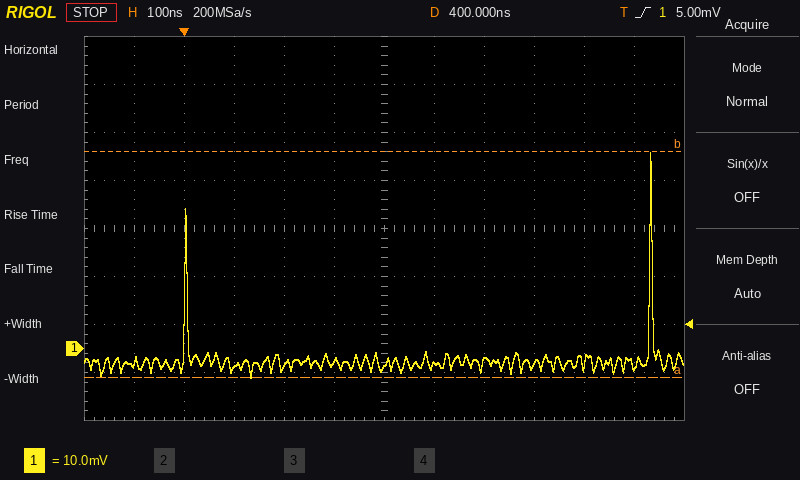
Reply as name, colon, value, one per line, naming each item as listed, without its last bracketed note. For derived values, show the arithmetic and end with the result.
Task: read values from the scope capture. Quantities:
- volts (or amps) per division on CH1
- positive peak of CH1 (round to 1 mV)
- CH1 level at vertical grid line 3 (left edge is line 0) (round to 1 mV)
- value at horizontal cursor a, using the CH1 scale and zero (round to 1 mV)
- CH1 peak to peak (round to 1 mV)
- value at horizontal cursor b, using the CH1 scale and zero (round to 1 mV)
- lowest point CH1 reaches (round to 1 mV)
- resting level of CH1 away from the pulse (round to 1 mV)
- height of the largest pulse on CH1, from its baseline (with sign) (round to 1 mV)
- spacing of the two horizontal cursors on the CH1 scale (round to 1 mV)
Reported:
volts (or amps) per division on CH1: 10 mV
positive peak of CH1: 41 mV
CH1 level at vertical grid line 3 (left edge is line 0): -4 mV
value at horizontal cursor a, using the CH1 scale and zero: -6 mV
CH1 peak to peak: 41 mV − (-6 mV) = 47 mV
value at horizontal cursor b, using the CH1 scale and zero: 41 mV
lowest point CH1 reaches: -6 mV
resting level of CH1 away from the pulse: -3 mV
height of the largest pulse on CH1, from its baseline (with sign): 41 mV − (-3 mV) = +44 mV
spacing of the two horizontal cursors on the CH1 scale: 47 mV
